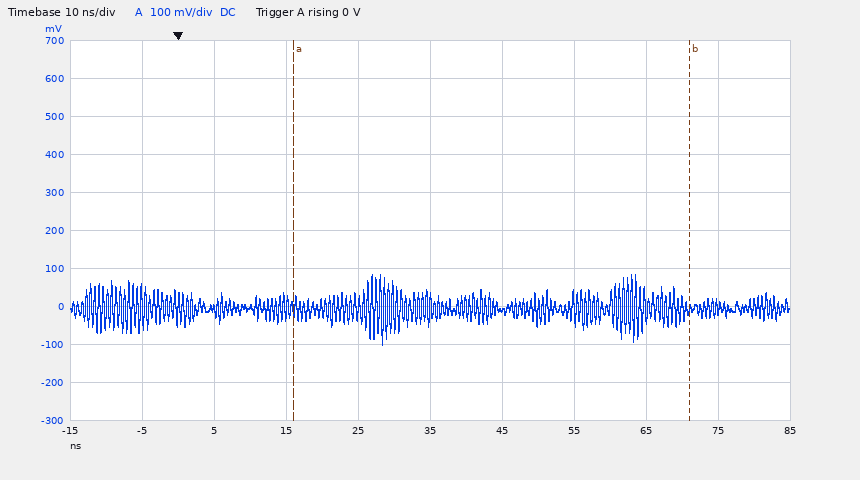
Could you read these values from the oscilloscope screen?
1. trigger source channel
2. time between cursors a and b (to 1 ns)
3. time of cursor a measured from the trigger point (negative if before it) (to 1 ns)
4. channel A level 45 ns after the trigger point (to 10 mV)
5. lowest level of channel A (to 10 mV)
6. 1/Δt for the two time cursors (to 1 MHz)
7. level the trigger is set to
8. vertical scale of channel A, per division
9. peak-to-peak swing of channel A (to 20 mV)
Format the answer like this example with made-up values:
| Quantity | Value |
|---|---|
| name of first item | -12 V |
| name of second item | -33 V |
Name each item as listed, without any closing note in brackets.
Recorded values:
| Quantity | Value |
|---|---|
| trigger source channel | channel A |
| time between cursors a and b | 55 ns |
| time of cursor a measured from the trigger point (negative if before it) | +16 ns |
| channel A level 45 ns after the trigger point | -10 mV |
| lowest level of channel A | -100 mV |
| 1/Δt for the two time cursors | 18 MHz |
| level the trigger is set to | 0 V |
| vertical scale of channel A, per division | 100 mV |
| peak-to-peak swing of channel A | 180 mV |
